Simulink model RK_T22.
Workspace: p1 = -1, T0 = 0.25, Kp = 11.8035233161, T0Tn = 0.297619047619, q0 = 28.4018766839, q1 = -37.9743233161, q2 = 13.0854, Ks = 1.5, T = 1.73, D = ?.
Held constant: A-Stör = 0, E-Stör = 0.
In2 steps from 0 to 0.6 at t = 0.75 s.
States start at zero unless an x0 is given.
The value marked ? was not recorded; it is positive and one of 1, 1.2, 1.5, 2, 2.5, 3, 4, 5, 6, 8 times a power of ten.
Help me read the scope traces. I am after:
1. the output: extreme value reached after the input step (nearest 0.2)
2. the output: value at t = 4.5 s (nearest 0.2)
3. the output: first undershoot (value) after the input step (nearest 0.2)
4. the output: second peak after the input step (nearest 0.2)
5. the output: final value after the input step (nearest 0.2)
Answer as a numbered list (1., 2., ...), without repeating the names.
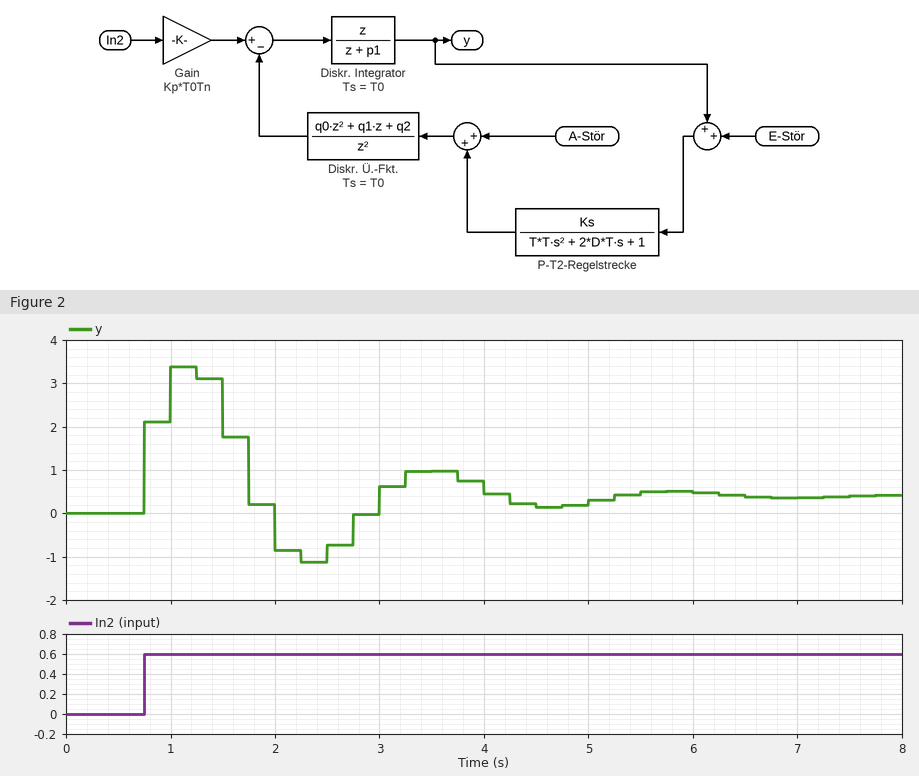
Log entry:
1. 3.4
2. 0.2
3. -1.2
4. 1.0
5. 0.4
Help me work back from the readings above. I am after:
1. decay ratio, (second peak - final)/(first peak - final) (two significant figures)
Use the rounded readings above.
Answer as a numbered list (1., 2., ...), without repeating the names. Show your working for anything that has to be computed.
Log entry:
1. (1 - 0.4) / (3.4 - 0.4) = 0.20
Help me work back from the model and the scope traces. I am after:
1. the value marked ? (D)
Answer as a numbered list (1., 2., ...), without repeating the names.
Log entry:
1. 1.2
